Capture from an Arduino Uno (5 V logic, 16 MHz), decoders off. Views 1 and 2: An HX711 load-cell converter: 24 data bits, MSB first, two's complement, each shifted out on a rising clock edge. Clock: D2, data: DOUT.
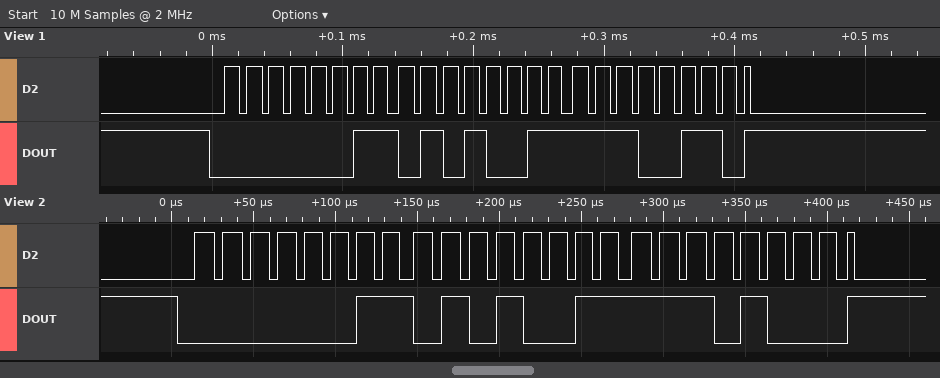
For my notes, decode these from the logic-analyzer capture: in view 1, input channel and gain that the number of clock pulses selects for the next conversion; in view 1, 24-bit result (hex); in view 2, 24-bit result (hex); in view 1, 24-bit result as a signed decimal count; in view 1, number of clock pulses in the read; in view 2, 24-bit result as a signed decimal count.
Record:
channel A, gain 128
0x0353E6
0x0353E8
218086
25
218088
